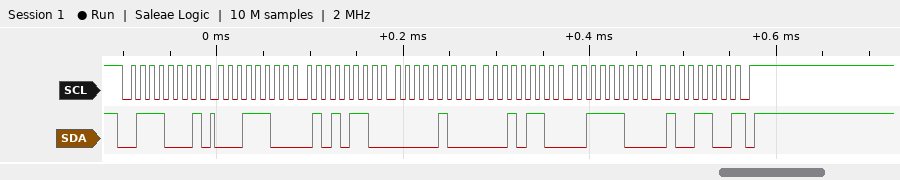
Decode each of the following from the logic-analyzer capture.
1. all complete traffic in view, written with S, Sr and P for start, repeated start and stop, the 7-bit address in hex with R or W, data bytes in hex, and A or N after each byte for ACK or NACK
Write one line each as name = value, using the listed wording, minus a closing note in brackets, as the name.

all complete traffic in view, written with S, Sr and P for start, repeated start and stop, the 7-bit address in hex with R or W, data bytes in hex, and A or N after each byte for ACK or NACK = S 38R A 1C A 56 A 04 A 16 A 3C A 4C N P
